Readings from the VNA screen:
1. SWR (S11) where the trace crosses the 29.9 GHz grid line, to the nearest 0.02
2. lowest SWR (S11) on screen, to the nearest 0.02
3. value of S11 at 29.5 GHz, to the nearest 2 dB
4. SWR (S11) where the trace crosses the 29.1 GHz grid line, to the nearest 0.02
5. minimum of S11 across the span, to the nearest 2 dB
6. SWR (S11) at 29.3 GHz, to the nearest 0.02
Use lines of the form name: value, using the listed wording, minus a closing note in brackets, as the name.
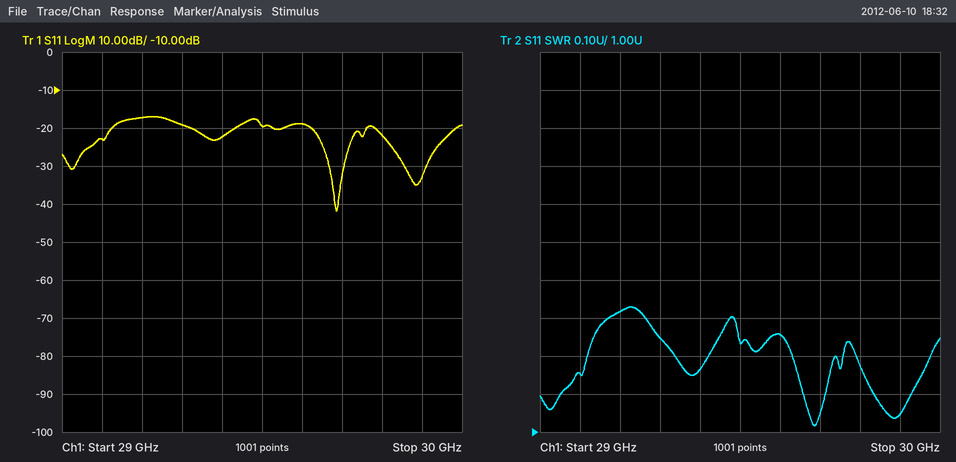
SWR (S11) where the trace crosses the 29.9 GHz grid line, to the nearest 0.02: 1.04
lowest SWR (S11) on screen, to the nearest 0.02: 1.02
value of S11 at 29.5 GHz, to the nearest 2 dB: -20 dB
SWR (S11) where the trace crosses the 29.1 GHz grid line, to the nearest 0.02: 1.16
minimum of S11 across the span, to the nearest 2 dB: -42 dB
SWR (S11) at 29.3 GHz, to the nearest 0.02: 1.24
